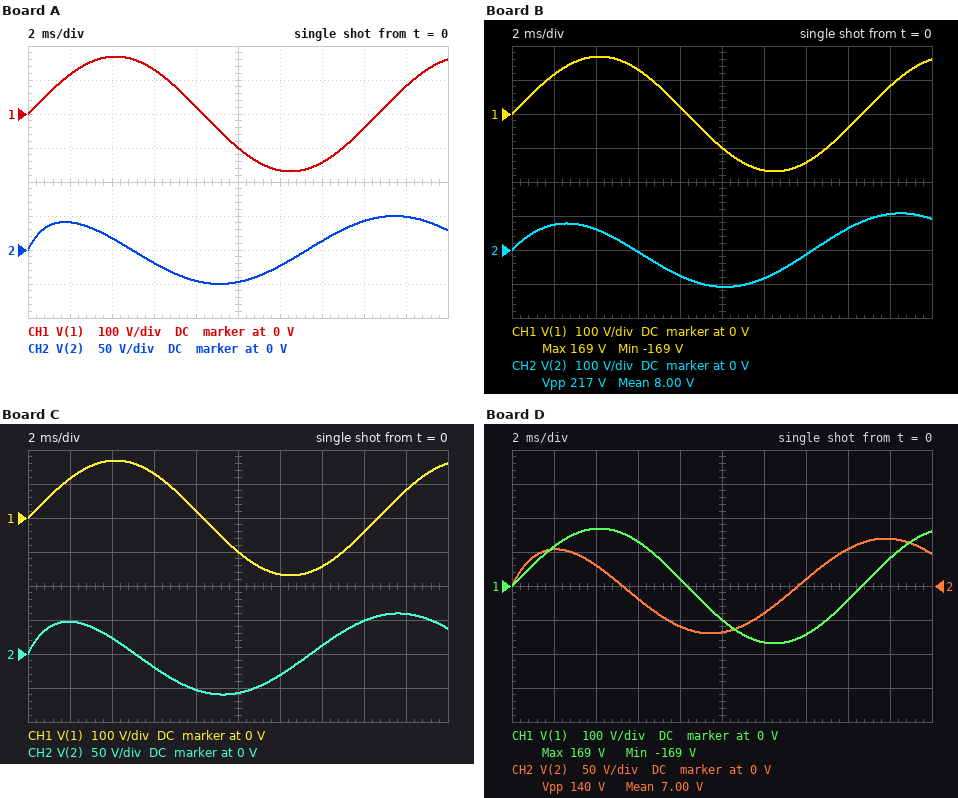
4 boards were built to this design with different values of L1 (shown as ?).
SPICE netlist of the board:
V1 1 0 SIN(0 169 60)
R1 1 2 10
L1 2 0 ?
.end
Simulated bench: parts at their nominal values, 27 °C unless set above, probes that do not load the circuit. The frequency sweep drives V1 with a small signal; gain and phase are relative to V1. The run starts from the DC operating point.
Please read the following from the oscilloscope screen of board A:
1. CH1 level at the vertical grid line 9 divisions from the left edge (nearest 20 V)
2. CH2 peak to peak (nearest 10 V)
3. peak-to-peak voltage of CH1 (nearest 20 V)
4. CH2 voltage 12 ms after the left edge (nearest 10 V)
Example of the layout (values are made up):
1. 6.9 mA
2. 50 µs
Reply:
1. 80 V
2. 100 V
3. 340 V
4. -20 V
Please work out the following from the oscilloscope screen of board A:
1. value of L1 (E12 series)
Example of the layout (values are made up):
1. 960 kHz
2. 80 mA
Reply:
1. 8.2 mH
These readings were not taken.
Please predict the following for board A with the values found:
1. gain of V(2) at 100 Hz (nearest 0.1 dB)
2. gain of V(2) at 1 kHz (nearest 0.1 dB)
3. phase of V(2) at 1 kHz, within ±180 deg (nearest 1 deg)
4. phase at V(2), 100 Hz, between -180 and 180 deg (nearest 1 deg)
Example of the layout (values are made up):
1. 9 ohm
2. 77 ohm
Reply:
1. -6.8 dB
2. -0.2 dB
3. 11 deg
4. 63 deg
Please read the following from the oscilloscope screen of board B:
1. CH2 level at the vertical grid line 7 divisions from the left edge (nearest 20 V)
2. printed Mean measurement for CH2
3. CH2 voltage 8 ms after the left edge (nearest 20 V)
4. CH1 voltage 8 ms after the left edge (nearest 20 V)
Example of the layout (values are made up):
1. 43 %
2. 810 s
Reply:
1. -20 V
2. 8.00 V
3. -80 V
4. 20 V
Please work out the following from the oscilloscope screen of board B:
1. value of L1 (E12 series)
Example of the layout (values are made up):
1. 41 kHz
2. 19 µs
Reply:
1. 22 mH
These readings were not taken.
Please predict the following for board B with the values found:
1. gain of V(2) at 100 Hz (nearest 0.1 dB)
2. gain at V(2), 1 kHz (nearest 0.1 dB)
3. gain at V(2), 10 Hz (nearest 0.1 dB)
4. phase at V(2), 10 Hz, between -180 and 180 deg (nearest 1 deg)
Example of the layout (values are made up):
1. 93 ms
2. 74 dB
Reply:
1. -1.8 dB
2. 0 dB
3. -17.3 dB
4. 82 deg
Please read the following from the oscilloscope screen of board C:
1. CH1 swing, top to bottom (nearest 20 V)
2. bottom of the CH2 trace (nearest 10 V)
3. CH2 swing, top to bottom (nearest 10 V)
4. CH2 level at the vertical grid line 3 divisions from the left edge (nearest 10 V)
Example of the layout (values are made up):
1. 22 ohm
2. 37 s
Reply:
1. 340 V
2. -60 V
3. 120 V
4. -20 V
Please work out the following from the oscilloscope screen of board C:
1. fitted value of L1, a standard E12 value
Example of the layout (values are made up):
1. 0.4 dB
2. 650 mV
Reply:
1. 10 mH
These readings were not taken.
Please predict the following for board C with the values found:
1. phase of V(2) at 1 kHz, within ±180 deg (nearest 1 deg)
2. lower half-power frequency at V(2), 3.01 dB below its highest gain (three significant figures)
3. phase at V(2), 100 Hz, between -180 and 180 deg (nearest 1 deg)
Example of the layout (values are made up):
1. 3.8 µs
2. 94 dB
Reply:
1. 9 deg
2. 159 Hz
3. 58 deg
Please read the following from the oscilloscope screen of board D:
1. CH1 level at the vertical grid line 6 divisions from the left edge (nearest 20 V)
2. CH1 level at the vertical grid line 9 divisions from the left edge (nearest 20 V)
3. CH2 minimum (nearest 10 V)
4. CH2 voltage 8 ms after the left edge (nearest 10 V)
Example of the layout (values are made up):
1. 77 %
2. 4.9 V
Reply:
1. -160 V
2. 80 V
3. -70 V
4. -60 V
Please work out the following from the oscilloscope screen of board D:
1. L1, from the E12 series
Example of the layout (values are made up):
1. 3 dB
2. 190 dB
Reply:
1. 12 mH
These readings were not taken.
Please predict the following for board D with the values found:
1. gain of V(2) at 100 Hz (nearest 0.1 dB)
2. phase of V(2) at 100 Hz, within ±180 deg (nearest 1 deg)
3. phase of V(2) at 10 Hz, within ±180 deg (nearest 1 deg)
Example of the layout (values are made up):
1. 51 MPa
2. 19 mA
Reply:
1. -4.4 dB
2. 53 deg
3. 86 deg
